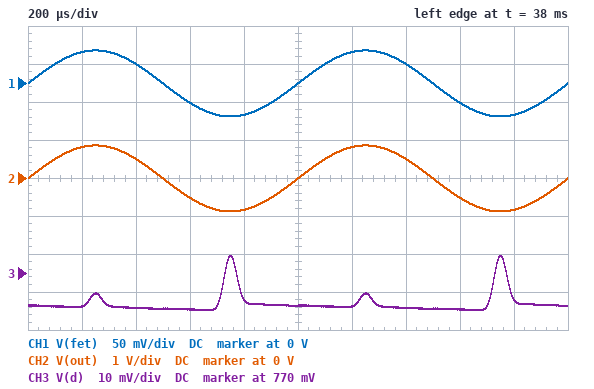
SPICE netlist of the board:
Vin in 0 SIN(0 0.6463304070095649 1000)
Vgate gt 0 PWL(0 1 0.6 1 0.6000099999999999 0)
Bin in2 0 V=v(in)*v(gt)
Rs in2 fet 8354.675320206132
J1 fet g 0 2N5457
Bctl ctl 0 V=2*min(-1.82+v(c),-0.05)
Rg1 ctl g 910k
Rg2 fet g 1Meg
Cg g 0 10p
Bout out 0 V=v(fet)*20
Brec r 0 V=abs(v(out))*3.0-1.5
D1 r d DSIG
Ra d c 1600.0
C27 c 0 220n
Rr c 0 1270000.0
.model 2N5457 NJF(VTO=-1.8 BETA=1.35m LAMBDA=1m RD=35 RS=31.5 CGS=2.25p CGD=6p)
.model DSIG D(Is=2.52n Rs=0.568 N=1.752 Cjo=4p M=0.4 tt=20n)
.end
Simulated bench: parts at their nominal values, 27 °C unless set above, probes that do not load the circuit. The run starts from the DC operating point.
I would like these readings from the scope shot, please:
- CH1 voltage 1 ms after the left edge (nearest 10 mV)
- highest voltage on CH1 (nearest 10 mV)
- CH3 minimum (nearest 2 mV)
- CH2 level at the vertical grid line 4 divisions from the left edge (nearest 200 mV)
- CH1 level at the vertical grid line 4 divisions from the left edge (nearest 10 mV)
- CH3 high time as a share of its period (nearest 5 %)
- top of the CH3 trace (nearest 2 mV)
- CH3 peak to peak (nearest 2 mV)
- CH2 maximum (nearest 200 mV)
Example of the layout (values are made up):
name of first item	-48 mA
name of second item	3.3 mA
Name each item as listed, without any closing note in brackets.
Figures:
CH1 voltage 1 ms after the left edge	0 V
highest voltage on CH1	40 mV
CH3 minimum	760 mV
CH2 level at the vertical grid line 4 divisions from the left edge	-800 mV
CH1 level at the vertical grid line 4 divisions from the left edge	-40 mV
CH3 high time as a share of its period	5 %
top of the CH3 trace	774 mV
CH3 peak to peak	14 mV
CH2 maximum	800 mV
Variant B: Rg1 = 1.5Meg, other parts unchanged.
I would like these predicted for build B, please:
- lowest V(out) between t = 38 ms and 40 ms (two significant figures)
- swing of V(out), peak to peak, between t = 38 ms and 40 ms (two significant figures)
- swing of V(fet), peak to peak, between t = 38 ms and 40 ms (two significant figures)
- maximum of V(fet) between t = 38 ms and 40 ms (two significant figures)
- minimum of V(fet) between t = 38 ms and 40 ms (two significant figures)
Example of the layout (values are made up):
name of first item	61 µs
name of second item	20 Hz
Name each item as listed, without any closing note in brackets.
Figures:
lowest V(out) between t = 38 ms and 40 ms	-800 mV
swing of V(out), peak to peak, between t = 38 ms and 40 ms	1.6 V
swing of V(fet), peak to peak, between t = 38 ms and 40 ms	79 mV
maximum of V(fet) between t = 38 ms and 40 ms	39 mV
minimum of V(fet) between t = 38 ms and 40 ms	-40 mV
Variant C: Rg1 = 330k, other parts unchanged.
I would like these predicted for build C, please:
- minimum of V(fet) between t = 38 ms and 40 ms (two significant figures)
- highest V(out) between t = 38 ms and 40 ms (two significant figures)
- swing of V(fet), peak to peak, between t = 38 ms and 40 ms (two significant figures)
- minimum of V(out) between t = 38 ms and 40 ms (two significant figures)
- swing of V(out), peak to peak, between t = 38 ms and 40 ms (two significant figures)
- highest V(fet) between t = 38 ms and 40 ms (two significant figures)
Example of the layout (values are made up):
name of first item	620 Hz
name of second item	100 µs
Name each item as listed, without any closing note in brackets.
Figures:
minimum of V(fet) between t = 38 ms and 40 ms	-48 mV
highest V(out) between t = 38 ms and 40 ms	970 mV
swing of V(fet), peak to peak, between t = 38 ms and 40 ms	97 mV
minimum of V(out) between t = 38 ms and 40 ms	-970 mV
swing of V(out), peak to peak, between t = 38 ms and 40 ms	1.9 V
highest V(fet) between t = 38 ms and 40 ms	48 mV
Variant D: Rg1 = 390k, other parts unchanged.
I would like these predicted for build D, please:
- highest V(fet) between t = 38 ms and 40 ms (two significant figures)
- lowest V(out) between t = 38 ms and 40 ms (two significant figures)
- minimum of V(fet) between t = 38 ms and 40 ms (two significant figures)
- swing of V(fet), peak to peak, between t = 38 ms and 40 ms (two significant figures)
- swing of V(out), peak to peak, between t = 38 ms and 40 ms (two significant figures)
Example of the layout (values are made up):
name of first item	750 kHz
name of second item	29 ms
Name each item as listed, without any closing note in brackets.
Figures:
highest V(fet) between t = 38 ms and 40 ms	48 mV
lowest V(out) between t = 38 ms and 40 ms	-960 mV
minimum of V(fet) between t = 38 ms and 40 ms	-48 mV
swing of V(fet), peak to peak, between t = 38 ms and 40 ms	96 mV
swing of V(out), peak to peak, between t = 38 ms and 40 ms	1.9 V
